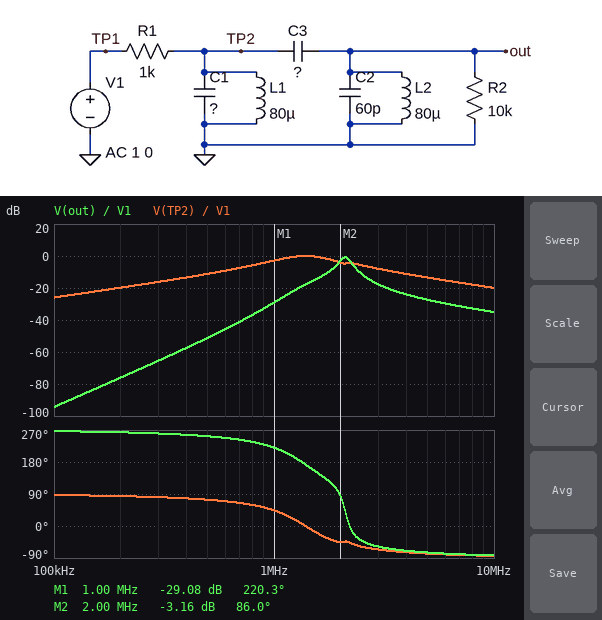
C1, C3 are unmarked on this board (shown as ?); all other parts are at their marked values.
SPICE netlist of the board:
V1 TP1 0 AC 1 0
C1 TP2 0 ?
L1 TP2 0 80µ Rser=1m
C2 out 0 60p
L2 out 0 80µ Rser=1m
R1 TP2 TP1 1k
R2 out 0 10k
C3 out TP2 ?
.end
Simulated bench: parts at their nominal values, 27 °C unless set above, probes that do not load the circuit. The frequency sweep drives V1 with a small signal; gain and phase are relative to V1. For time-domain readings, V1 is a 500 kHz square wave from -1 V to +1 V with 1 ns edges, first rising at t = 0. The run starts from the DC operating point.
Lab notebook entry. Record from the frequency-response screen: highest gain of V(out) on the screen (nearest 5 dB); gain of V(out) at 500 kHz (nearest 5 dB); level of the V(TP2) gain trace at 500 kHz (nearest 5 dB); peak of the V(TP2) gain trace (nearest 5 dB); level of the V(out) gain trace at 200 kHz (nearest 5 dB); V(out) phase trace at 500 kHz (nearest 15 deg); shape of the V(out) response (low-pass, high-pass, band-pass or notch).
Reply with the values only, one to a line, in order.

0 dB
-50 dB
-10 dB
0 dB
-75 dB
255 deg
band-pass
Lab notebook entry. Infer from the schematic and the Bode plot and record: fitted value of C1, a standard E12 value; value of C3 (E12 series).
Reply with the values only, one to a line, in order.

150 pF
12 pF
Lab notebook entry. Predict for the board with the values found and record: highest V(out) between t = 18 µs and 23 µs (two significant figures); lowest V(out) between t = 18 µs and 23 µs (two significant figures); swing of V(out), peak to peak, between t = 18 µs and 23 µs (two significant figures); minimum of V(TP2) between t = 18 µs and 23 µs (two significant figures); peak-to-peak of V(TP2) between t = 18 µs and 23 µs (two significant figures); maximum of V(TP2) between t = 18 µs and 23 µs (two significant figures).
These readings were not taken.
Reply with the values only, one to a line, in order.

130 mV
-130 mV
260 mV
-890 mV
1.8 V
890 mV
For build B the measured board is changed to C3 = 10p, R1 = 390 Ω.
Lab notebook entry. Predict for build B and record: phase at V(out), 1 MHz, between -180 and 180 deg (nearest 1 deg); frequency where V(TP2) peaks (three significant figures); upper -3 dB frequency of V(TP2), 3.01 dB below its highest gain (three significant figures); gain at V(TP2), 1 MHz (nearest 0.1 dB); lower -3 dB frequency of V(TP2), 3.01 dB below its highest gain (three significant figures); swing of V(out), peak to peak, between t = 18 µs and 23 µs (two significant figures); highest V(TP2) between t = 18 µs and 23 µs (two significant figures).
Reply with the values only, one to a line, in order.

-163 deg
1.40 MHz
3.21 MHz
-0.6 dB
623 kHz
290 mV
1.4 V
